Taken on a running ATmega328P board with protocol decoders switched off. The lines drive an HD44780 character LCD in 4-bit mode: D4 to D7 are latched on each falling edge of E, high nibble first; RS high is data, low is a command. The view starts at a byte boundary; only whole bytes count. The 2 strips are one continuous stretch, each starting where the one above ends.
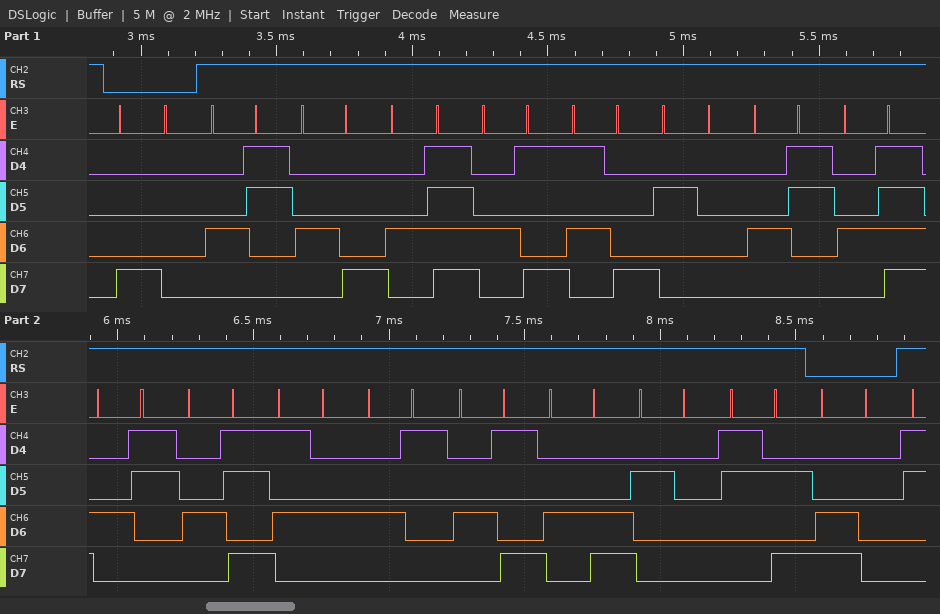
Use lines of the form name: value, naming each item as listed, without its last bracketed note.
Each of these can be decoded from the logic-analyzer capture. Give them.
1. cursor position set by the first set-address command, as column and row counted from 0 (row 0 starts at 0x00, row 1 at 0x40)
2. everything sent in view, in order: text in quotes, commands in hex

cursor position set by the first set-address command, as column and row counted from 0: column 0, row 0
everything sent in view, in order: text in quotes, commands in hex: 0x80 "CHOIX COCKTAIL :" 0xC0
